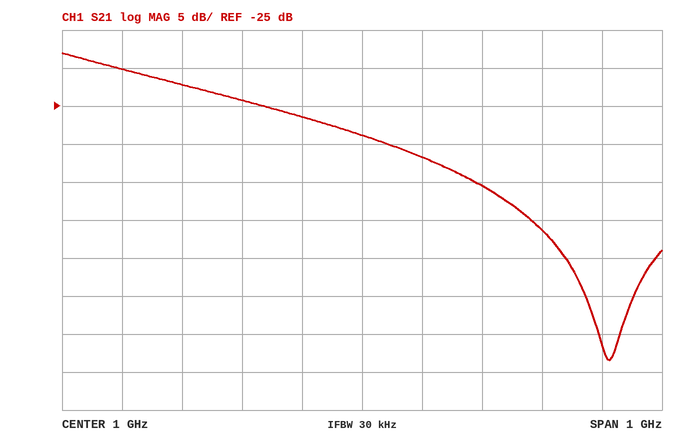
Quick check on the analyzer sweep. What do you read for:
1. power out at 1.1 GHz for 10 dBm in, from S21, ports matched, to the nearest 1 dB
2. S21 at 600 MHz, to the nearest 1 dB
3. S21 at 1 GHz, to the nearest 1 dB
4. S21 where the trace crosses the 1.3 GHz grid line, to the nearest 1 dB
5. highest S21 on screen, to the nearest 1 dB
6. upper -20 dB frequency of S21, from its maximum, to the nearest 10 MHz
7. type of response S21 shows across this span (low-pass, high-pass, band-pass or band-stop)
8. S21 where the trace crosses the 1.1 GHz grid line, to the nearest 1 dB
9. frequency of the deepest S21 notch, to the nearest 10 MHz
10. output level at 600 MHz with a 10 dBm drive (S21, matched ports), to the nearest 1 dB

-22 dBm
-20 dB
-29 dB
-41 dB
-18 dB
1.25 GHz
low-pass
-32 dB
1.41 GHz
-10 dBm
